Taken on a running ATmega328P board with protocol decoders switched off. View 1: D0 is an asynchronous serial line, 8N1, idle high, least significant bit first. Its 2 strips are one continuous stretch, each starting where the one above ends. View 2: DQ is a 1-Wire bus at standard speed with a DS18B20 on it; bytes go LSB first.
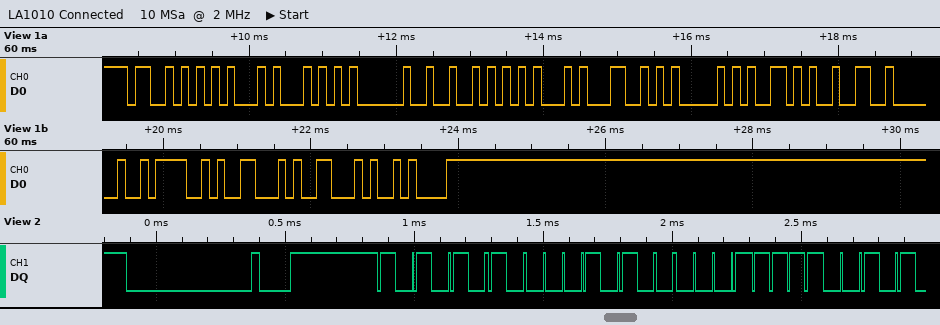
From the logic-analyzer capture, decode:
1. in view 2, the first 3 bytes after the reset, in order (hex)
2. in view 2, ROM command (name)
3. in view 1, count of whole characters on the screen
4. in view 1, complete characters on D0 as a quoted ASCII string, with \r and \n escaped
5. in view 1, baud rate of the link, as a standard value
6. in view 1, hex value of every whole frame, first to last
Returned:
55 28 F8
Match ROM
15
"SET RELAY2 OFF\n"
9600 baud
0x53 0x45 0x54 0x20 0x52 0x45 0x4C 0x41 0x59 0x32 0x20 0x4F 0x46 0x46 0x0A
